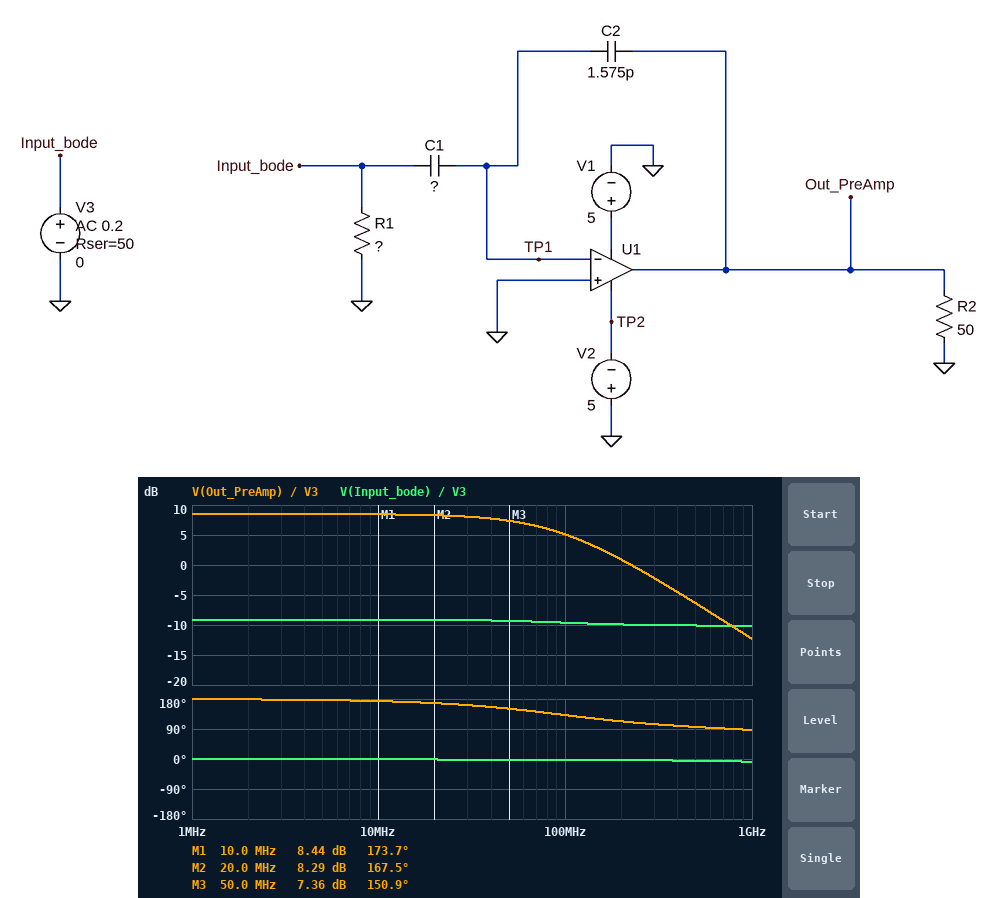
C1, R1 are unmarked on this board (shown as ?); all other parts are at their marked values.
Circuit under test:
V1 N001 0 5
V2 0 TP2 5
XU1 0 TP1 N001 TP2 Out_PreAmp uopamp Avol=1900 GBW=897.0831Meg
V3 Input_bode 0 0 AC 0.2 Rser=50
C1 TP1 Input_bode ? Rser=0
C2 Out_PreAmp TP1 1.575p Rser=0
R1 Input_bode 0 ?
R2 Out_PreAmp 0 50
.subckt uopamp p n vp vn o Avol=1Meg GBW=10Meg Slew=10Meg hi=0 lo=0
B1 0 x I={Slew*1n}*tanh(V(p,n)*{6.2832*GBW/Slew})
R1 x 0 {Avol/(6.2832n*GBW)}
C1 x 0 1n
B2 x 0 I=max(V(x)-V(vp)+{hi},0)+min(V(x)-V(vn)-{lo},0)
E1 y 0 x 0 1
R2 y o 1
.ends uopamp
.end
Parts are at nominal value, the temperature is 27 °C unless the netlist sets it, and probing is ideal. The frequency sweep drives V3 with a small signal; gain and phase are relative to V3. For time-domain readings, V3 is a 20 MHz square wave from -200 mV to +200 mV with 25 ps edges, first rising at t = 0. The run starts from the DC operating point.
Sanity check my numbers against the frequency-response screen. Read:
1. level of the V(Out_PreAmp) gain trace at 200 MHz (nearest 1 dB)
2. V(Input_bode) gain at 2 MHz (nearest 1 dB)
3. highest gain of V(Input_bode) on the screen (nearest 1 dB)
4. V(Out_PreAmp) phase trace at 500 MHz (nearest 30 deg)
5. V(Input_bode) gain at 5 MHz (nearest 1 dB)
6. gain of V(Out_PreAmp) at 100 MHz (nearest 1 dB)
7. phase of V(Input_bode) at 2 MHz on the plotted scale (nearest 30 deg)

1 dB
-9 dB
-9 dB
90 deg
-9 dB
5 dB
0 deg
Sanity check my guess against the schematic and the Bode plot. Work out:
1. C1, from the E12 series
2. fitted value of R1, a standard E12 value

12 pF
27 Ω
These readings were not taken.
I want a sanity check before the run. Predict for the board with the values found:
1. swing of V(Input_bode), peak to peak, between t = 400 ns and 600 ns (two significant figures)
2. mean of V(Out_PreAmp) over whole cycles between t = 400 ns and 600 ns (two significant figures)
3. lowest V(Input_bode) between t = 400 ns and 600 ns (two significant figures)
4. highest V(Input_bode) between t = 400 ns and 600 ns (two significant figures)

140 mV
-120 mV
-70 mV
70 mV
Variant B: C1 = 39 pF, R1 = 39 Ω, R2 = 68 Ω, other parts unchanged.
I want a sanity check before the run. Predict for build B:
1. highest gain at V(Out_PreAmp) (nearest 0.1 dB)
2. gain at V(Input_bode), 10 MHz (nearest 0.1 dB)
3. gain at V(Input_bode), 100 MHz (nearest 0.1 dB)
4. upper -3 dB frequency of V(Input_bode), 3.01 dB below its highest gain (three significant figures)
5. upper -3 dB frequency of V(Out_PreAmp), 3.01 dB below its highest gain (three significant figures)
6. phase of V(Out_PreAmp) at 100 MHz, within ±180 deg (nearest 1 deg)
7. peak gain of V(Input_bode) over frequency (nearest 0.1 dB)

20.6 dB
-7.3 dB
-8.5 dB
3.60 GHz
29.5 MHz
105 deg
-7.2 dB
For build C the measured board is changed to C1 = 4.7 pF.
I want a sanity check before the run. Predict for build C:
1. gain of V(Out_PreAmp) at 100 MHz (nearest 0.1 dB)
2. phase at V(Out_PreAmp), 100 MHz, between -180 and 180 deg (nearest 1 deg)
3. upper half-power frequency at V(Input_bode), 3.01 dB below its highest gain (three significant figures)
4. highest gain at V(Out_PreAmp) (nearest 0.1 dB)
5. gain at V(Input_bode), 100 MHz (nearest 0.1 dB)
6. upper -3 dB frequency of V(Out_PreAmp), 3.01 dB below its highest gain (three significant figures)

-0.6 dB
153 deg
6.59 GHz
0.4 dB
-9.2 dB
204 MHz
